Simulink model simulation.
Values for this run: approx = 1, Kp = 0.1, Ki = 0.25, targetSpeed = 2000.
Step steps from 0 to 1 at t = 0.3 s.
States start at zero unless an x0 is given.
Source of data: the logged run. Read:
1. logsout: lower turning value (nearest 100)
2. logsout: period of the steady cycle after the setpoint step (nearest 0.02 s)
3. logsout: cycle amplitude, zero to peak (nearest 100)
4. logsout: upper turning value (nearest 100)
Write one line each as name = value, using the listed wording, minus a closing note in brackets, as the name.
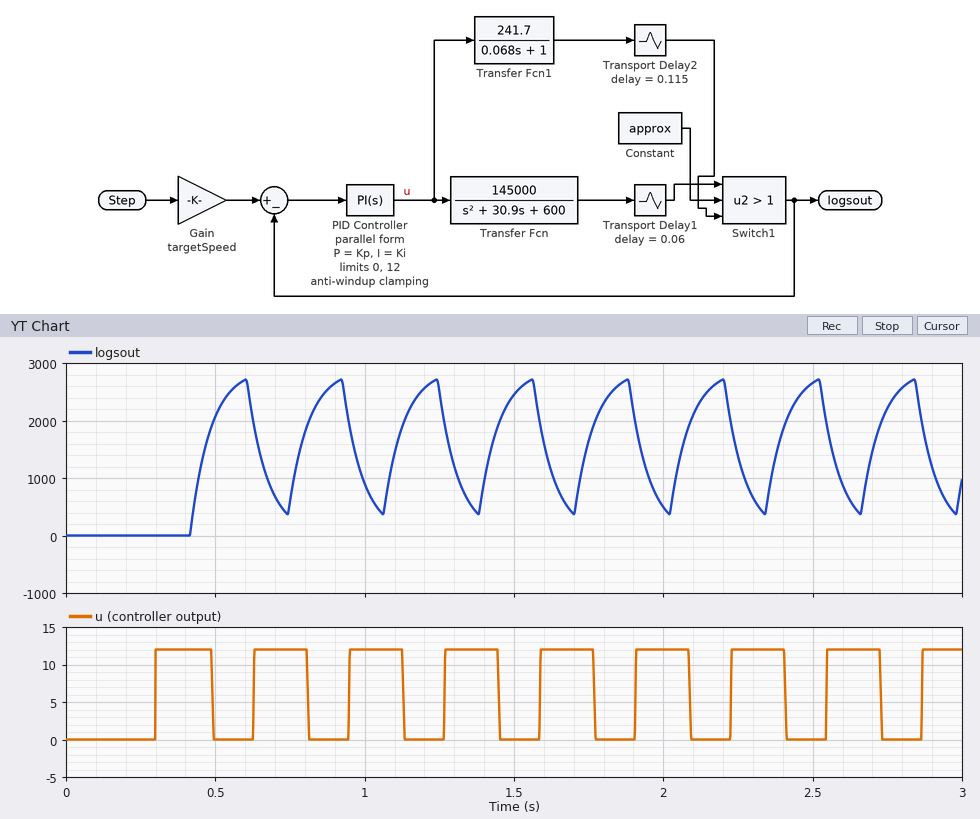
logsout: lower turning value = 400
logsout: period of the steady cycle after the setpoint step = 0.32 s
logsout: cycle amplitude, zero to peak = 1200
logsout: upper turning value = 2700
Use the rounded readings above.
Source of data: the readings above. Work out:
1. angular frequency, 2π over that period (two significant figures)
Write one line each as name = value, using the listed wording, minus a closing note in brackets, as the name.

angular frequency, 2π over that period = 20 rad/s
